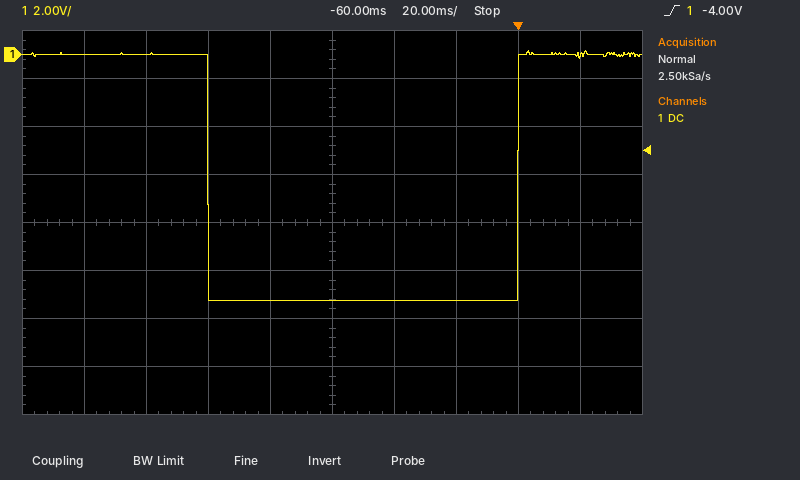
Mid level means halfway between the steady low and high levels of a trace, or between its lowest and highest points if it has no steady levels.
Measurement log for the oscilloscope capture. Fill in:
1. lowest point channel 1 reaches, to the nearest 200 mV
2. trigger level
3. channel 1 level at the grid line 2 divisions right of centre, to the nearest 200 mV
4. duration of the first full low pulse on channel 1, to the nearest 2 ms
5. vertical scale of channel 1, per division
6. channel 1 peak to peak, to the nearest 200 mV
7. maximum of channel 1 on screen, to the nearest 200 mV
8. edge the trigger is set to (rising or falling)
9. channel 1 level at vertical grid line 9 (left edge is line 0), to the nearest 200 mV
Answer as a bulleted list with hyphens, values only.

- -10.2 V
- -4.00 V
- -10.2 V
- 100 ms
- 2 V
- 10.4 V
- 200 mV
- rising
- 0.0 V
